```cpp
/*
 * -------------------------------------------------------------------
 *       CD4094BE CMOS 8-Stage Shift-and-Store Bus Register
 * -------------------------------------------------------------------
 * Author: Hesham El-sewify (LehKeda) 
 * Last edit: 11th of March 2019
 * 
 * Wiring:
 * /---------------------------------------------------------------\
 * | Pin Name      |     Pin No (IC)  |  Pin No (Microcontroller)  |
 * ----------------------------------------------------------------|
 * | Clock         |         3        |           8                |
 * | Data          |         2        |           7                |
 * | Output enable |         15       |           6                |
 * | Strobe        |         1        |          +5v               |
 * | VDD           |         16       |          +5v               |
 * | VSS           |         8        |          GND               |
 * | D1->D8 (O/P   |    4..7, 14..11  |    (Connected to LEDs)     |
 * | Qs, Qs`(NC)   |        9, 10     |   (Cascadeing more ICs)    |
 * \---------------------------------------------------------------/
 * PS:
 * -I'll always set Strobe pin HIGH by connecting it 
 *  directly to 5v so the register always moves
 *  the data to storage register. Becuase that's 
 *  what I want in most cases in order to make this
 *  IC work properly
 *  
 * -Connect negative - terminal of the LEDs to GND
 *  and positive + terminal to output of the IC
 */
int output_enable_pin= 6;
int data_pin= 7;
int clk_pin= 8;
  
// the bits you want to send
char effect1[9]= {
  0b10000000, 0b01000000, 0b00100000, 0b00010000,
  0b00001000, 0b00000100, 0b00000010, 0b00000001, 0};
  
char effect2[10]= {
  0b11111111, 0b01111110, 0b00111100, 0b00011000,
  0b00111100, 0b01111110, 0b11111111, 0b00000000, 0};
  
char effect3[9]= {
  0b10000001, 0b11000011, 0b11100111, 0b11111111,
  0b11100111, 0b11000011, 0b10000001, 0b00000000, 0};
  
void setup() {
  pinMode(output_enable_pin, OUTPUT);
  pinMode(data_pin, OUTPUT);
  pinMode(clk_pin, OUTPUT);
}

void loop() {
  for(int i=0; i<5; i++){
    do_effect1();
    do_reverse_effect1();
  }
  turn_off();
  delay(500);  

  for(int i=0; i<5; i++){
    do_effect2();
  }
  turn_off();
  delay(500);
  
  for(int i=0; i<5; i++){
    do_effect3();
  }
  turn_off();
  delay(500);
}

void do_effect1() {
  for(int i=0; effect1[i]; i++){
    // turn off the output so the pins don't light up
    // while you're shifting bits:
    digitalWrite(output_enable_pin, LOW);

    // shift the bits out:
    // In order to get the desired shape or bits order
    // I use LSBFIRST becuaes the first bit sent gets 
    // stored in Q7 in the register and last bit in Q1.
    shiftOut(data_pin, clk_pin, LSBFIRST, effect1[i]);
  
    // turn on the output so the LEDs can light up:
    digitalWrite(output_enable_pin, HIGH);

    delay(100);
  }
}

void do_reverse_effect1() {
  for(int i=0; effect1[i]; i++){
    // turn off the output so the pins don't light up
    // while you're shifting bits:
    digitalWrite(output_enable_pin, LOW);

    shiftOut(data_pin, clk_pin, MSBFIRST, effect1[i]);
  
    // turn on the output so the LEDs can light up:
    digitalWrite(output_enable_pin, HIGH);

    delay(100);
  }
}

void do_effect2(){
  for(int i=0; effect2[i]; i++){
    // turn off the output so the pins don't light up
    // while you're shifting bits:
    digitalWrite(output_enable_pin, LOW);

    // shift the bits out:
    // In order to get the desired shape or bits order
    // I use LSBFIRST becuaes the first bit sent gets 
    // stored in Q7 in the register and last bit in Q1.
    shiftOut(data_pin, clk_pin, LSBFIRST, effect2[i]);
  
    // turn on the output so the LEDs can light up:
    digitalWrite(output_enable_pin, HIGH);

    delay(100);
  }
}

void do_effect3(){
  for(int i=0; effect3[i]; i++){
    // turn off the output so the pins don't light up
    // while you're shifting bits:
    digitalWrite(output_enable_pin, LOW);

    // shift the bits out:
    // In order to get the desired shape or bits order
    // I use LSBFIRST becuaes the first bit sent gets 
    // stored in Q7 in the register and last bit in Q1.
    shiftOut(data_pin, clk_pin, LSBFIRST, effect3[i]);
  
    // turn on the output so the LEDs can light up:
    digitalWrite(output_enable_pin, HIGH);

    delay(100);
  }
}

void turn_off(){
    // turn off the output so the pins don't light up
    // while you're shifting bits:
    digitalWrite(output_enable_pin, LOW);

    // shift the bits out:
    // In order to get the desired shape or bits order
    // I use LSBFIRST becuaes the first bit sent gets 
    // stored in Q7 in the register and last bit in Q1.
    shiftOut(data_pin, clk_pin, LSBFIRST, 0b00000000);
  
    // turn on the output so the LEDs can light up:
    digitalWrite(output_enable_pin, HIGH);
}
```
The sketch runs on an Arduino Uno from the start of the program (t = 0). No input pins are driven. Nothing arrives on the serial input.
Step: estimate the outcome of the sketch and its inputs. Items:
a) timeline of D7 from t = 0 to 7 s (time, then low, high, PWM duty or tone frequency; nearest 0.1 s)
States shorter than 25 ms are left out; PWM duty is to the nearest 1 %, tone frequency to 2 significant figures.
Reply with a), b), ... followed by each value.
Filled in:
a) 0 s high; 0.1 s low; 1.5 s high; 1.7 s low; 3.1 s high; 3.3 s low; 4.7 s high; 4.9 s low; 6.3 s high; 6.5 s low
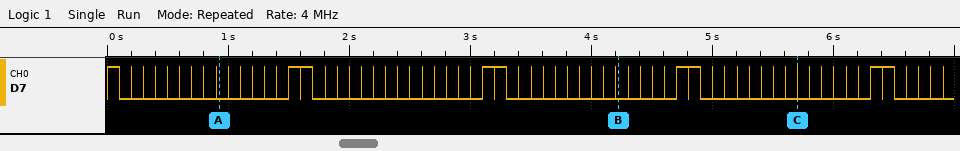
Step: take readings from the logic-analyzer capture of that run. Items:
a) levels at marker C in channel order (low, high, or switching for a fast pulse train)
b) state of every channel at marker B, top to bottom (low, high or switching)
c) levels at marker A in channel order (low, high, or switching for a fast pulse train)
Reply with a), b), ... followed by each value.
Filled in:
a) D7 low
b) D7 low
c) D7 low
